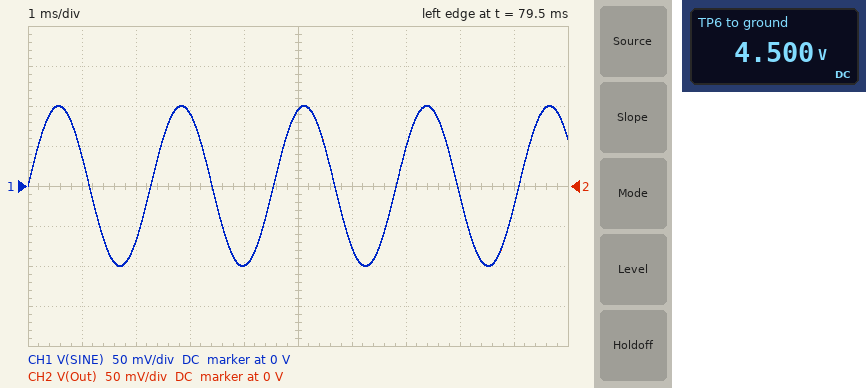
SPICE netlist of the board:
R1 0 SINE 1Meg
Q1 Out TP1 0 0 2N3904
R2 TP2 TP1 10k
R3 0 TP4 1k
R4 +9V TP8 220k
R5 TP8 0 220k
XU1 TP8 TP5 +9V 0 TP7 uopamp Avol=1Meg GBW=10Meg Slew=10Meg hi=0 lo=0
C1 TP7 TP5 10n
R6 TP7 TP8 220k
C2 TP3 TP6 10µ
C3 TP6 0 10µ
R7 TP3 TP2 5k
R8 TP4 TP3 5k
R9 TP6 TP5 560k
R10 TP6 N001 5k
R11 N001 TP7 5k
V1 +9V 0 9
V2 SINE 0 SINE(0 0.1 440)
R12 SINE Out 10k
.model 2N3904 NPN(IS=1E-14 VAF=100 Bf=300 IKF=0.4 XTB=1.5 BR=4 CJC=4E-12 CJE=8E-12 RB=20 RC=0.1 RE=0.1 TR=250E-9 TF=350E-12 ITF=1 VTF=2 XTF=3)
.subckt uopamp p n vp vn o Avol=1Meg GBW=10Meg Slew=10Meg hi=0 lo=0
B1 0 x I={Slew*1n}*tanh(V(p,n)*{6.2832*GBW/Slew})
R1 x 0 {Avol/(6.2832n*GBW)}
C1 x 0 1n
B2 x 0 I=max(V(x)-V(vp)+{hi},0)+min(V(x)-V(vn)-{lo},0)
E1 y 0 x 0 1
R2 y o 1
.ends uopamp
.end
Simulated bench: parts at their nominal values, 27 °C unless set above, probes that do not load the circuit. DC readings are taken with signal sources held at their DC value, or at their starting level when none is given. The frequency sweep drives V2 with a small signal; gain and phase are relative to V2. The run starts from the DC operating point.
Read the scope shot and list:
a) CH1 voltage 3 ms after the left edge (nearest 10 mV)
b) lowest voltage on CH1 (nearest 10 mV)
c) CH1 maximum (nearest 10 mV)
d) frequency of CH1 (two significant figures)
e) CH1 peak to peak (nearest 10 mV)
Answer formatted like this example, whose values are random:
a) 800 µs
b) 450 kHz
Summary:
a) 90 mV
b) -100 mV
c) 100 mV
d) 440 Hz
e) 200 mV
